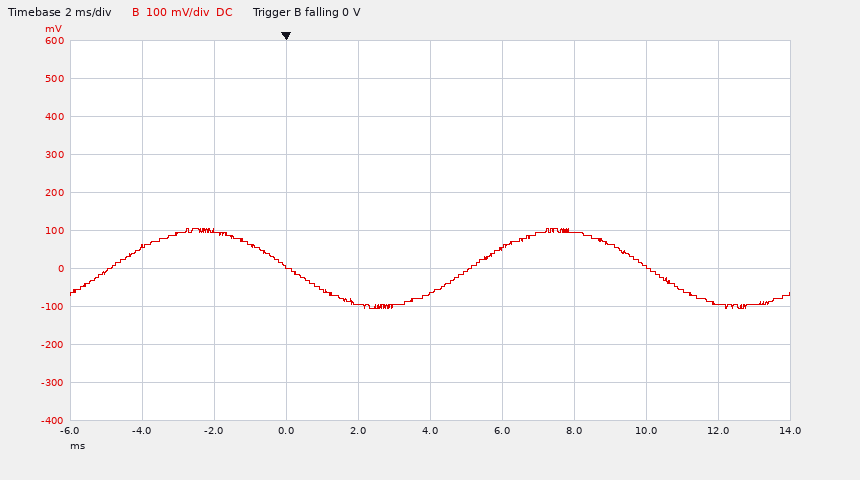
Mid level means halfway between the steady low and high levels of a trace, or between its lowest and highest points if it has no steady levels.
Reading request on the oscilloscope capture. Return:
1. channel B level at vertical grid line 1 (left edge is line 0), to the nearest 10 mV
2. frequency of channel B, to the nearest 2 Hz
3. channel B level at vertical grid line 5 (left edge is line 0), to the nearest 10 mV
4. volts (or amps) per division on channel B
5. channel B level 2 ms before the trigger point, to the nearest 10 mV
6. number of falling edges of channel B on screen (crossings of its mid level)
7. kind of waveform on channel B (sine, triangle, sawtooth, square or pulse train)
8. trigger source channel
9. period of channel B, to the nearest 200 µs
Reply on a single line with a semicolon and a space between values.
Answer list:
60 mV; 100 Hz; -70 mV; 100 mV; 100 mV; 2; sine; channel B; 10.0 ms
